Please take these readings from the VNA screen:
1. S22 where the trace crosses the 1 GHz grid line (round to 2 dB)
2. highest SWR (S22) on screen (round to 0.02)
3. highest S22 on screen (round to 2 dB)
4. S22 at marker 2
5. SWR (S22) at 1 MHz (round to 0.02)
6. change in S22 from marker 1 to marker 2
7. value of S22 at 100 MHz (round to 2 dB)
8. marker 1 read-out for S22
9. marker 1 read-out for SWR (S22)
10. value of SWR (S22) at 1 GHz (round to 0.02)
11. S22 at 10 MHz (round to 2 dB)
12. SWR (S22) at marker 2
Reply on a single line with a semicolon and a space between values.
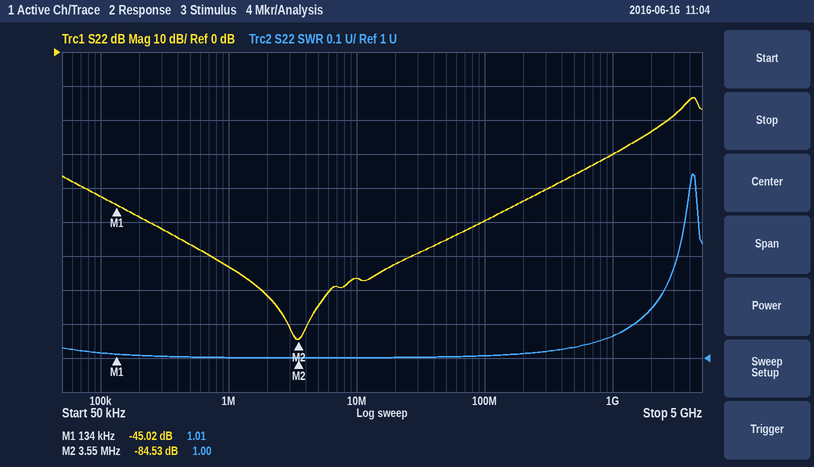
-30 dB; 1.54; -14 dB; -84.53 dB; 1.00; -39.51 dB; -50 dB; -45.02 dB; 1.01; 1.06; -66 dB; 1.00
